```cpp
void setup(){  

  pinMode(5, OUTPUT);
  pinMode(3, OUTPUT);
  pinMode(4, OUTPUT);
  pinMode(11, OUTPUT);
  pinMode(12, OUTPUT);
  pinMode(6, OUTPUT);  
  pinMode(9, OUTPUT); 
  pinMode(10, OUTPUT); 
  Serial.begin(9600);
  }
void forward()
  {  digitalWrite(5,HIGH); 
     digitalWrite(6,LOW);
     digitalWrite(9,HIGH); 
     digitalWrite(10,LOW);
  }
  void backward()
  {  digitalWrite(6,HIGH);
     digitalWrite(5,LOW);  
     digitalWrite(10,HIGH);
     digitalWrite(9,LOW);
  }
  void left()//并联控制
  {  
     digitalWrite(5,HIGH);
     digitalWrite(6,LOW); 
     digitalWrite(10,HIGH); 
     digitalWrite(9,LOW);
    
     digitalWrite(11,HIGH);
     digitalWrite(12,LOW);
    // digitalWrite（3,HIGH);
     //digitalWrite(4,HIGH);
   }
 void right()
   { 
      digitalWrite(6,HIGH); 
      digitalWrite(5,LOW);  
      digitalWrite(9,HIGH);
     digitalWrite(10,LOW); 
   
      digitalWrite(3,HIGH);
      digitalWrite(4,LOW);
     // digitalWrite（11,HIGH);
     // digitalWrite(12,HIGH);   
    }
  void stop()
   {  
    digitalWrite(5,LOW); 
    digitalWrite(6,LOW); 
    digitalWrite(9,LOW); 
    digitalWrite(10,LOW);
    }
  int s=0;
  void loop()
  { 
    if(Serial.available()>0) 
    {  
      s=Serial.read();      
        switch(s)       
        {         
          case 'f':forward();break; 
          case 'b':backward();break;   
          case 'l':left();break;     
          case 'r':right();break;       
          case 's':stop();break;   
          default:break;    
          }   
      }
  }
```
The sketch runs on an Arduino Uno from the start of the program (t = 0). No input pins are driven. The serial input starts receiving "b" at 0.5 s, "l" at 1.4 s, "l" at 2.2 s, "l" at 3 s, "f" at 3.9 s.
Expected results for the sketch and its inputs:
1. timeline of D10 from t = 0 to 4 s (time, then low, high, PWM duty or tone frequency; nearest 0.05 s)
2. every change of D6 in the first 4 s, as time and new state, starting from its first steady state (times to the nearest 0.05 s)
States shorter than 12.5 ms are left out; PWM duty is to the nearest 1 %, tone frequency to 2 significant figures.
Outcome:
0 s low; 0.5 s high; 3.9 s low
0 s low; 0.5 s high; 1.4 s low
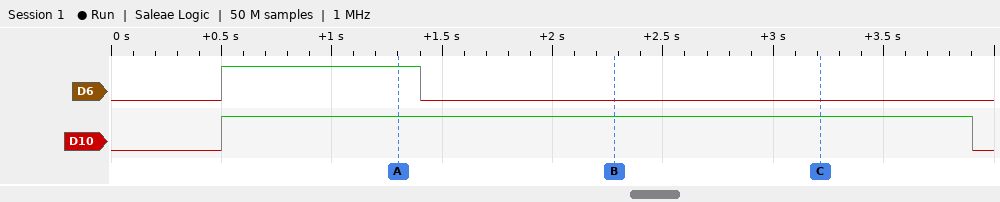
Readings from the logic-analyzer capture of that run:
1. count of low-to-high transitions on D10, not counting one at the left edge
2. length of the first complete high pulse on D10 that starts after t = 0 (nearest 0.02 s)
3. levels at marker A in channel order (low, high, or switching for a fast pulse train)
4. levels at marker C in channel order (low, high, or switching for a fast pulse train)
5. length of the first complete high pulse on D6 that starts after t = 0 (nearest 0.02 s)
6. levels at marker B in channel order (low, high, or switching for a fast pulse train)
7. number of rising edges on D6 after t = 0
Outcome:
1
3.40 s
D6 high, D10 high
D6 low, D10 high
0.90 s
D6 low, D10 high
1
